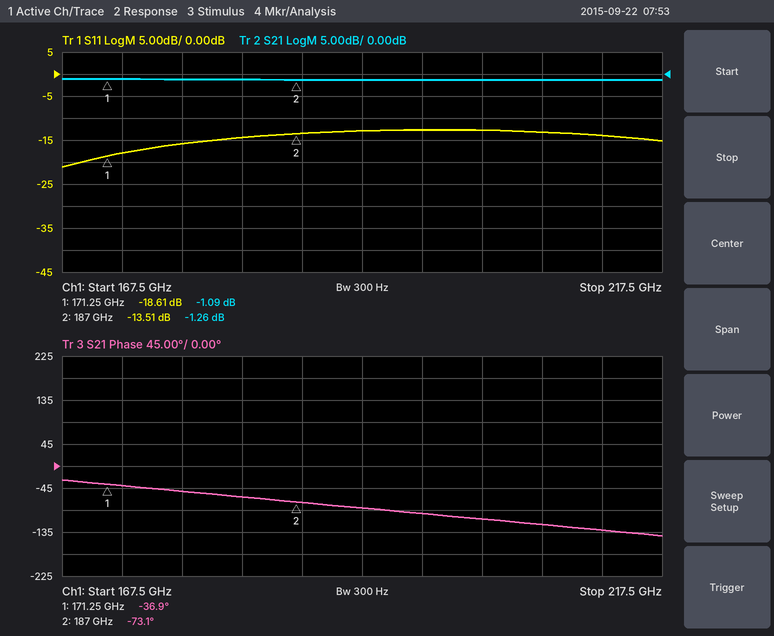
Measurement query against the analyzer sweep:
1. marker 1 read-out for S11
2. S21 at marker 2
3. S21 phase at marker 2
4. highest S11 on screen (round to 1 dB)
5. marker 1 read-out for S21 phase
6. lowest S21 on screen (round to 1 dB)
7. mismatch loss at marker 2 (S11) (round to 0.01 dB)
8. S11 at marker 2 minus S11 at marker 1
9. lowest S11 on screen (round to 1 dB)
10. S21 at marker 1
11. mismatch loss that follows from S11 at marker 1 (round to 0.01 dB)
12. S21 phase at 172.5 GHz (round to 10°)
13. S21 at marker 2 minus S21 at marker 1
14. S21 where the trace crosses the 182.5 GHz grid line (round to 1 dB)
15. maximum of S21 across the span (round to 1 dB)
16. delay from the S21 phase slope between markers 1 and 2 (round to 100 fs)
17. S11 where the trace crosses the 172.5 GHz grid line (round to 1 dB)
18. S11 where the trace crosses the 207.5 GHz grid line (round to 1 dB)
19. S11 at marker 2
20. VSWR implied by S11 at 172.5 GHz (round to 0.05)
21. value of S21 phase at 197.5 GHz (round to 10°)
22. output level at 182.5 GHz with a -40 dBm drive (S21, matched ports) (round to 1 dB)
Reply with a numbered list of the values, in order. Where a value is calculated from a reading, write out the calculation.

1. -18.61 dB
2. -1.26 dB
3. -73.1°
4. -13 dB
5. -36.9°
6. -1 dB
7. −10 log10(1 − 10^(-13.51/10)) ≈ 0.20 dB
8. -13.51 − (-18.61) = 5.10 dB
9. -21 dB
10. -1.09 dB
11. −10 log10(1 − 10^(-18.61/10)) ≈ 0.06 dB
12. -40°
13. -1.26 − (-1.09) = -0.17 dB
14. -1 dB
15. -1 dB
16. −(-73.1° − (-36.9°))/(360° × 15.75 GHz) ≈ 6.4 ps
17. -18 dB
18. -13 dB
19. -13.51 dB
20. |Γ| = 10^(-18/20) = 0.1259; VSWR = (1 + 0.1259)/(1 − 0.1259) ≈ 1.29, so 1.30 to the nearest 0.05
21. -100°
22. -40 dBm + (-1 dB) = -41 dBm
